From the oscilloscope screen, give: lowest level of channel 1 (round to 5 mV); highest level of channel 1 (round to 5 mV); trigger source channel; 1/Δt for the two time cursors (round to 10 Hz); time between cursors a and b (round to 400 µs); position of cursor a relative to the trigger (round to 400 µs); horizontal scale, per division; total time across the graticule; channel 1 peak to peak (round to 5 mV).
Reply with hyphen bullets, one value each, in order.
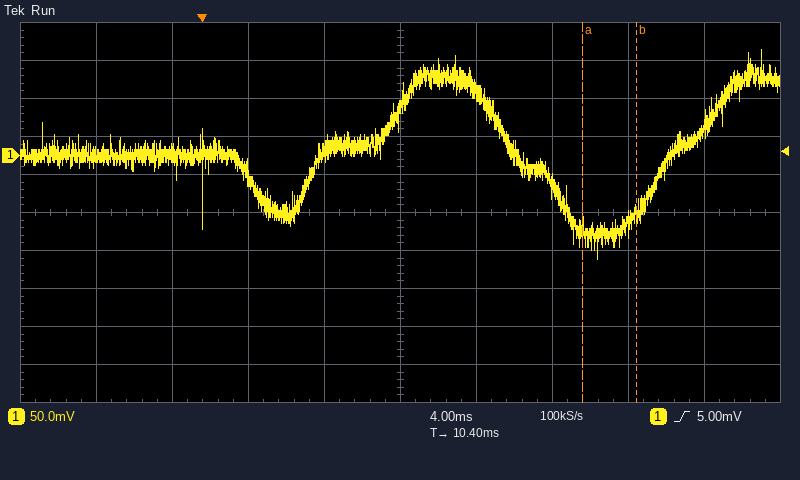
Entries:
- -135 mV
- 140 mV
- channel 1
- 360 Hz
- 2.8 ms
- +20.0 ms
- 4 ms
- 40 ms
- 275 mV
